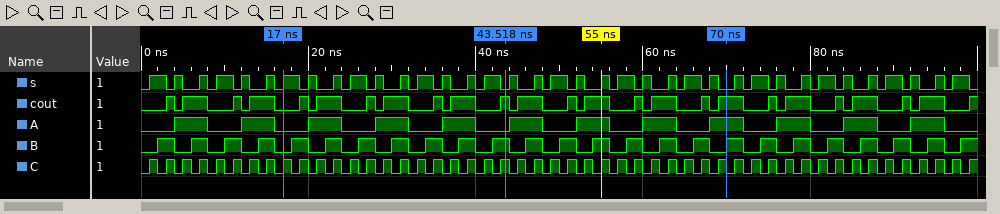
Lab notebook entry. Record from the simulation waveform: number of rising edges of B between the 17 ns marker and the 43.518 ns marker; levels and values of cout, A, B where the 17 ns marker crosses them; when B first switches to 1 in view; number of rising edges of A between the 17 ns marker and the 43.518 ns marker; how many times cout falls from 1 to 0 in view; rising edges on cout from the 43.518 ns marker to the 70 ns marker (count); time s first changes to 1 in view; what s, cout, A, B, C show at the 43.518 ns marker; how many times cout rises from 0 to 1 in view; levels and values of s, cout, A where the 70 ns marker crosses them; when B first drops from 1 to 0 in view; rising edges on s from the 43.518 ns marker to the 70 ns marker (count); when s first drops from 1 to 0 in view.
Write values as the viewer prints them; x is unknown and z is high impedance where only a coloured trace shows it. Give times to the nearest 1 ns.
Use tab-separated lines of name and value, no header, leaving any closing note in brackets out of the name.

number of rising edges of B between the 17 ns marker and the 43.518 ns marker	7
levels and values of cout, A, B where the 17 ns marker crosses them	cout=0, A=0, B=0
when B first switches to 1 in view	2 ns
number of rising edges of A between the 17 ns marker and the 43.518 ns marker	3
how many times cout falls from 1 to 0 in view	24
rising edges on cout from the 43.518 ns marker to the 70 ns marker	7
time s first changes to 1 in view	1 ns
what s, cout, A, B, C show at the 43.518 ns marker	s=0, cout=1, A=0, B=1, C=1
how many times cout rises from 0 to 1 in view	25
levels and values of s, cout, A where the 70 ns marker crosses them	s=0, cout=1, A=1
when B first drops from 1 to 0 in view	4 ns
rising edges on s from the 43.518 ns marker to the 70 ns marker	10
when s first drops from 1 to 0 in view	3 ns
